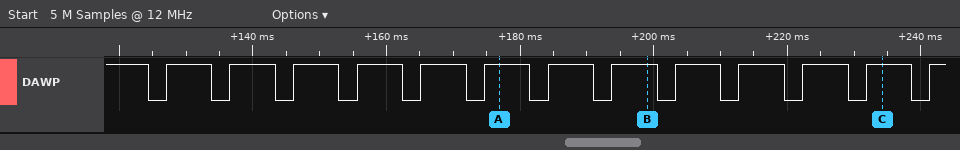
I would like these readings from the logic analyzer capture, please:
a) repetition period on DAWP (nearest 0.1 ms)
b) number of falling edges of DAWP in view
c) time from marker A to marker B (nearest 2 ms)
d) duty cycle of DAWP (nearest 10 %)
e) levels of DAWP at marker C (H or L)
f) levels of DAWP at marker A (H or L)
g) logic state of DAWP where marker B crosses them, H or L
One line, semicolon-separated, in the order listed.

9.5 ms; 13; 22 ms; 70 %; DAWP=H; DAWP=H; DAWP=H
